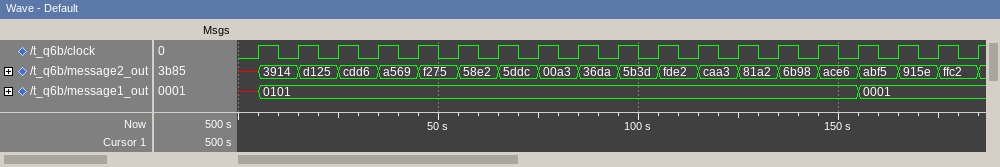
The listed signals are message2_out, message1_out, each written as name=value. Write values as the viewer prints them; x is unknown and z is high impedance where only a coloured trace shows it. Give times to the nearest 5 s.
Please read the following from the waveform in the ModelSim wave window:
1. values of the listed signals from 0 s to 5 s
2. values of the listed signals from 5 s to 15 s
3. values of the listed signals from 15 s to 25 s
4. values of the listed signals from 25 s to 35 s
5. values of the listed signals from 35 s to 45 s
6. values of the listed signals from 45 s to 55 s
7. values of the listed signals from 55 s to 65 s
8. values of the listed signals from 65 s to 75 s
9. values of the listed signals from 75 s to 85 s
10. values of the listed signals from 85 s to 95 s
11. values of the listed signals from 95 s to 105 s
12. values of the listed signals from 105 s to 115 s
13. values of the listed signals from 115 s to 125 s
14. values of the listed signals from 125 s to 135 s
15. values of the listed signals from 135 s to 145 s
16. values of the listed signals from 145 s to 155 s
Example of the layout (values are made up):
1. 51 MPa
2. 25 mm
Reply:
1. message2_out=x, message1_out=x
2. message2_out=3914, message1_out=0101
3. message2_out=d125, message1_out=0101
4. message2_out=cdd6, message1_out=0101
5. message2_out=a569, message1_out=0101
6. message2_out=f275, message1_out=0101
7. message2_out=58e2, message1_out=0101
8. message2_out=5ddc, message1_out=0101
9. message2_out=00a3, message1_out=0101
10. message2_out=36da, message1_out=0101
11. message2_out=5b3d, message1_out=0101
12. message2_out=fde2, message1_out=0101
13. message2_out=caa3, message1_out=0101
14. message2_out=81a2, message1_out=0101
15. message2_out=6b98, message1_out=0101
16. message2_out=ace6, message1_out=0101
